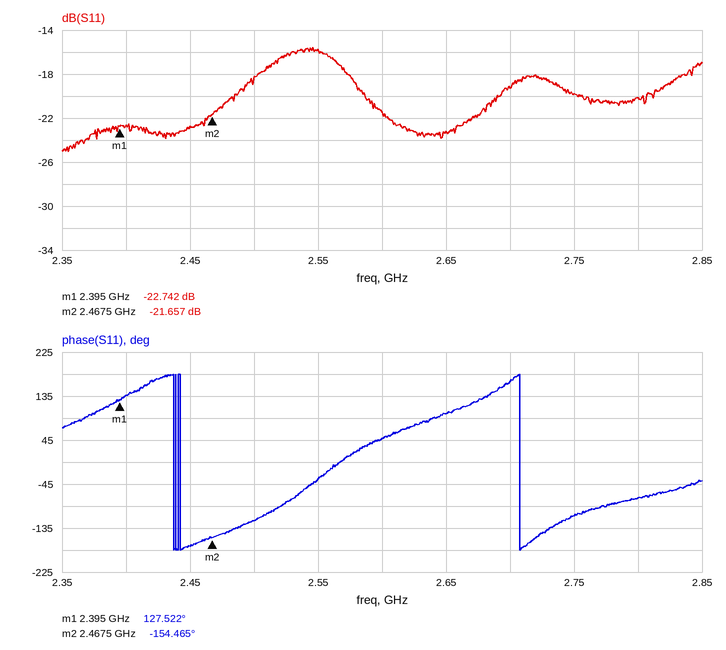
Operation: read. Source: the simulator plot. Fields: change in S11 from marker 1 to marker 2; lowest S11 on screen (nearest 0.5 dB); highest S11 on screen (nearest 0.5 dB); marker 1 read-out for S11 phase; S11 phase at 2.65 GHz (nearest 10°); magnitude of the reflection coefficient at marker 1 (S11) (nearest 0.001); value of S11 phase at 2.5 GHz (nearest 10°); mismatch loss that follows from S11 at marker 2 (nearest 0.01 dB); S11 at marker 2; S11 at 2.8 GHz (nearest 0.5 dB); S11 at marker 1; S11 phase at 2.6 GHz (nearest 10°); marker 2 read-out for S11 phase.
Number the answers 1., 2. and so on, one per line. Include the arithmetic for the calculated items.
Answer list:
1. -21.657 − (-22.742) = 1.085 dB
2. -25.0 dB
3. -15.5 dB
4. 127.522°
5. 100°
6. 10^(-22.742/20) ≈ 0.073
7. -120°
8. −10 log10(1 − 10^(-21.657/10)) ≈ 0.03 dB
9. -21.657 dB
10. -20.0 dB
11. -22.742 dB
12. 50°
13. -154.465°
